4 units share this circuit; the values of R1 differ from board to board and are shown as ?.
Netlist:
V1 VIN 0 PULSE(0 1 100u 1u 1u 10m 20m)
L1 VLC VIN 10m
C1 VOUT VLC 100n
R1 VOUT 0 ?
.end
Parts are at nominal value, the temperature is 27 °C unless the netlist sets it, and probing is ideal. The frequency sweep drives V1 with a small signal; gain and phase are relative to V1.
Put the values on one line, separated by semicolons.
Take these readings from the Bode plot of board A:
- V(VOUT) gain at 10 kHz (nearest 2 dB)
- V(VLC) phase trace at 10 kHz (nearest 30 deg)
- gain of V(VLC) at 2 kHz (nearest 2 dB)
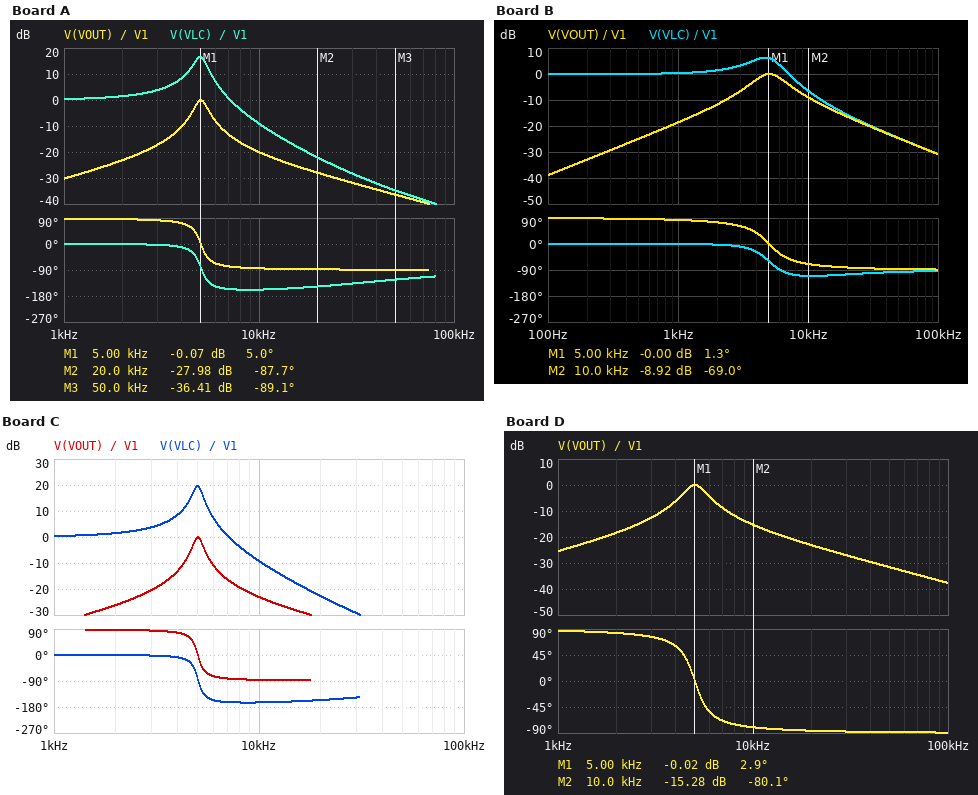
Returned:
-20 dB; -150 deg; 2 dB
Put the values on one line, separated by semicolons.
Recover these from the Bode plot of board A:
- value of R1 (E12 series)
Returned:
47 Ω
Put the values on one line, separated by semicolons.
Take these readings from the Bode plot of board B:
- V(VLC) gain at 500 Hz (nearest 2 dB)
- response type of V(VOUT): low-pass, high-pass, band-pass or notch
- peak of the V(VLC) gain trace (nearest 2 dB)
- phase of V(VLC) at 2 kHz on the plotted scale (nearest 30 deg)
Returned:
0 dB; band-pass; 6 dB; 0 deg
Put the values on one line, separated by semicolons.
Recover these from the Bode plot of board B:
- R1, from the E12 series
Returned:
180 Ω
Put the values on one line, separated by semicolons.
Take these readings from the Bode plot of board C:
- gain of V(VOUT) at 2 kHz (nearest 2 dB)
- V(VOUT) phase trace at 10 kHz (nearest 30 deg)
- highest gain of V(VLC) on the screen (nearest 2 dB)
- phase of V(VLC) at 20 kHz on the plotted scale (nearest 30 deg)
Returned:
-26 dB; -90 deg; 20 dB; -150 deg
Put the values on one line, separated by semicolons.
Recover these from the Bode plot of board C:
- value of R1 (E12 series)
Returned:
33 Ω
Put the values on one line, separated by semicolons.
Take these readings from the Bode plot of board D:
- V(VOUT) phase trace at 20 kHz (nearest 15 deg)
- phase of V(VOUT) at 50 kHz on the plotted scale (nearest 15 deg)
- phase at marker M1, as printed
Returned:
-90 deg; -90 deg; 2.9 deg
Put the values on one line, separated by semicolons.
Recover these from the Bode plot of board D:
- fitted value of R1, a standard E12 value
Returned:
82 Ω
